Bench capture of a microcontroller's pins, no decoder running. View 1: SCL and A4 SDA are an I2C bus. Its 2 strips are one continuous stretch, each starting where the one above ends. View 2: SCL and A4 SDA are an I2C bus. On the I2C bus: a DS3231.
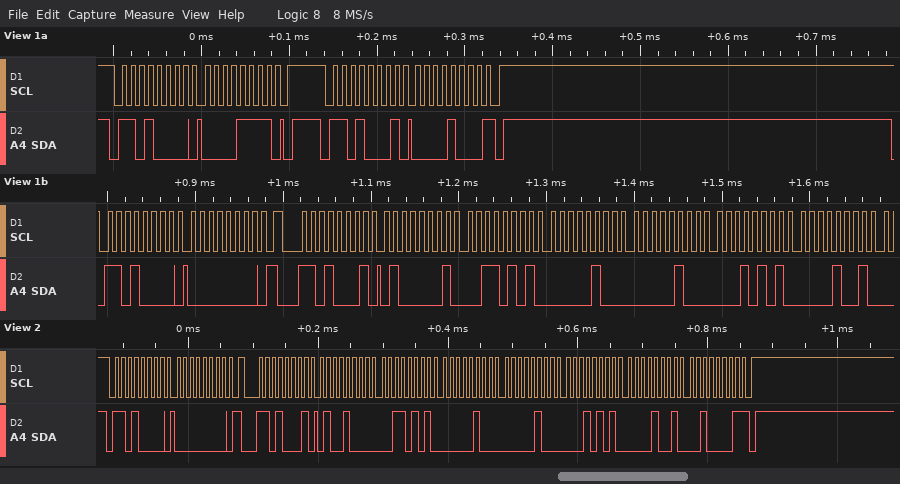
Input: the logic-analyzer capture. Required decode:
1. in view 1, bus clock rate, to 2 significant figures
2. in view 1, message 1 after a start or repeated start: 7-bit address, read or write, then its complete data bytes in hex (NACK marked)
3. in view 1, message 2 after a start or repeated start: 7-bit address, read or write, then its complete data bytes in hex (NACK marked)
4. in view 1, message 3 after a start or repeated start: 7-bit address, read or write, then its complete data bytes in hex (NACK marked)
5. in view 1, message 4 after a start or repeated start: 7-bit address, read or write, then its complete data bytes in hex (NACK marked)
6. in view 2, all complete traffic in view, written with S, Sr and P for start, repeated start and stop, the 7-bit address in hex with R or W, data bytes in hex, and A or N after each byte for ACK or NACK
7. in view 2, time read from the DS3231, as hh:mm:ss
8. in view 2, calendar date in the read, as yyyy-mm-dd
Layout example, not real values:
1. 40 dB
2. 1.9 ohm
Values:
1. 100 kHz
2. 0x68 write: 0F
3. 0x68 read: 08 NACK
4. 0x68 write: 00
5. 0x68 read: 41 35 04 04 15 09
6. S 68W A 00 A Sr 68R A 48 A 35 A 04 A 04 A 15 A 09 A 21 N P
7. 04:35:48
8. 2021-09-15
